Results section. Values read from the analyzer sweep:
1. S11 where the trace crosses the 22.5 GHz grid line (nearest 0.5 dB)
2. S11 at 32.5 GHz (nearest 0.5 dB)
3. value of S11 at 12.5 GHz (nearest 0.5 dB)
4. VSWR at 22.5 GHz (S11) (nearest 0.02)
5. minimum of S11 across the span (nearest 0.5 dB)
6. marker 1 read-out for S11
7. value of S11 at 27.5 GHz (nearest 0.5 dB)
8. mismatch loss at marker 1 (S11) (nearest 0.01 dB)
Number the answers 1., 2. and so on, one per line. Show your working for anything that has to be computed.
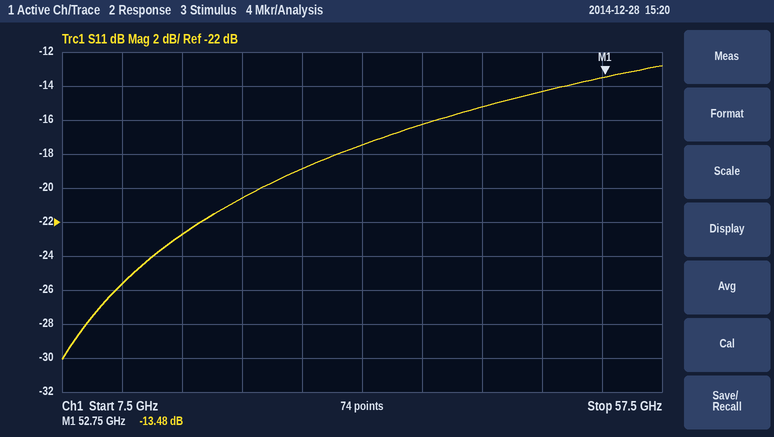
1. -20.5 dB
2. -17.5 dB
3. -25.5 dB
4. |Γ| = 10^(-20.5/20) = 0.0944; VSWR = (1 + 0.0944)/(1 − 0.0944) ≈ 1.21, so 1.20 to the nearest 0.02
5. -30.0 dB
6. -13.48 dB
7. -19.0 dB
8. −10 log10(1 − 10^(-13.48/10)) ≈ 0.20 dB
